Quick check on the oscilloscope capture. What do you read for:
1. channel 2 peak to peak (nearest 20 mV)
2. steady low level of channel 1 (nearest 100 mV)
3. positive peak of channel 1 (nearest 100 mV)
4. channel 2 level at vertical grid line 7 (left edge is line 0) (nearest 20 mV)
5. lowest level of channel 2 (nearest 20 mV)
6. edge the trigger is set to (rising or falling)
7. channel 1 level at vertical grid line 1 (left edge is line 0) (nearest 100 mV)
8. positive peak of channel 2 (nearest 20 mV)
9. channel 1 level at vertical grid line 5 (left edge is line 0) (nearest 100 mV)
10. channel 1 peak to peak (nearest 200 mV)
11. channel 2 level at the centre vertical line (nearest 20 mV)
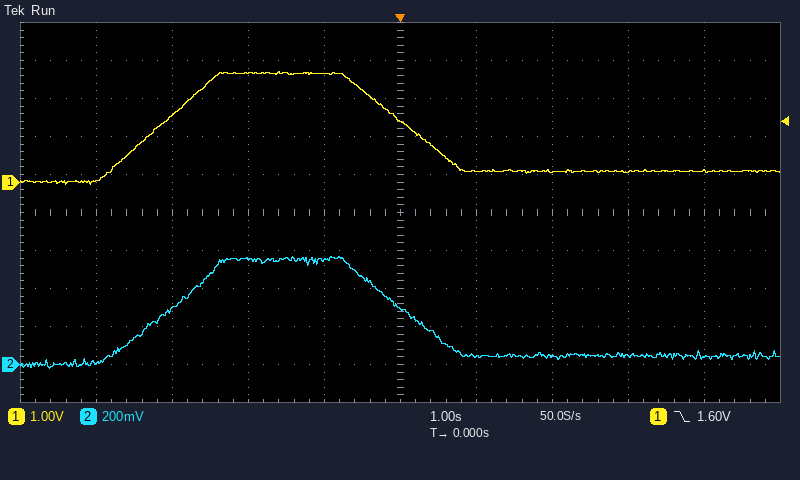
580 mV
300 mV
2.9 V
40 mV
-20 mV
falling
0.0 V
560 mV
1.6 V
3.0 V
300 mV
